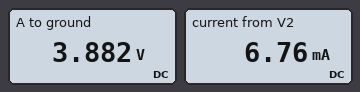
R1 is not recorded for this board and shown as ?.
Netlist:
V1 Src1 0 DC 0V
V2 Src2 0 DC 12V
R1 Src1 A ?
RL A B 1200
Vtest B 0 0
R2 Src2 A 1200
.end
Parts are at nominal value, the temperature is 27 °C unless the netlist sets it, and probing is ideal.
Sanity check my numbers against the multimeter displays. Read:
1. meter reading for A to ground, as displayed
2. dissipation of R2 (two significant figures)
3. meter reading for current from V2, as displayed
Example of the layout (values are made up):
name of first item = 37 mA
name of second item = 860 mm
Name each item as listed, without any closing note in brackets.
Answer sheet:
meter reading for A to ground, as displayed = 3.882 V
dissipation of R2 = 55 mW
meter reading for current from V2, as displayed = 6.76 mA
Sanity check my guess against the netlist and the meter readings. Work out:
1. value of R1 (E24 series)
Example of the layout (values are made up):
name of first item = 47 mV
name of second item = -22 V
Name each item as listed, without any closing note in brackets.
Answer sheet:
value of R1 = 1.1 kΩ
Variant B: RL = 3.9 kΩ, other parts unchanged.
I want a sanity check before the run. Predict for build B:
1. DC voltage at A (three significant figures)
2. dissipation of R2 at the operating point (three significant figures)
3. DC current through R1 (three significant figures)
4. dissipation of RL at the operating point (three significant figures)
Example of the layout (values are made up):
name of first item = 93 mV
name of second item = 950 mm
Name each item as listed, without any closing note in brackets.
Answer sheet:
DC voltage at A = 5.00 V
dissipation of R2 at the operating point = 40.8 mW
DC current through R1 = 4.55 mA
dissipation of RL at the operating point = 6.42 mW
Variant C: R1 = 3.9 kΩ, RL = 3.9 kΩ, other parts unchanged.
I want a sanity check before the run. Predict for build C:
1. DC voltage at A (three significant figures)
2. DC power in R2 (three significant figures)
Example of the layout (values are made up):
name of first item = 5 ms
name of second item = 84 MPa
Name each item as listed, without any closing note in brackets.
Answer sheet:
DC voltage at A = 7.43 V
DC power in R2 = 17.4 mW
